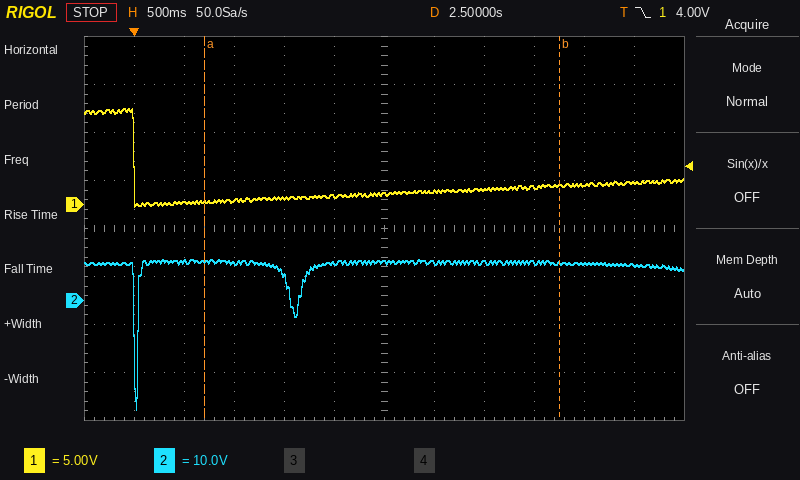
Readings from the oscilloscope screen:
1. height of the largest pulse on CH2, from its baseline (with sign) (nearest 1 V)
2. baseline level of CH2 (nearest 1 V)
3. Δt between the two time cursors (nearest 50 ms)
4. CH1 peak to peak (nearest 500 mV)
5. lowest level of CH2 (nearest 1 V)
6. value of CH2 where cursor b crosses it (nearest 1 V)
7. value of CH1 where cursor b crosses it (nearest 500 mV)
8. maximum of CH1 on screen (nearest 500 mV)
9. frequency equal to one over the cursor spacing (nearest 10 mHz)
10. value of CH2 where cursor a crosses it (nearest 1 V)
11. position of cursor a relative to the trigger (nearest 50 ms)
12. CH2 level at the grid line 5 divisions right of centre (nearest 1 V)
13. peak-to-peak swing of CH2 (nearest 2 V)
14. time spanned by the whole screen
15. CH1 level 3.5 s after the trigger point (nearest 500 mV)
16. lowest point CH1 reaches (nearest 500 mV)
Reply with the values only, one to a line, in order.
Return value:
-31 V
8 V
3.55 s
10.0 V
-23 V
8 V
2.0 V
10.0 V
280 mHz
8 V
+700 ms
7 V
32 V
6 s
1.5 V
0.0 V
